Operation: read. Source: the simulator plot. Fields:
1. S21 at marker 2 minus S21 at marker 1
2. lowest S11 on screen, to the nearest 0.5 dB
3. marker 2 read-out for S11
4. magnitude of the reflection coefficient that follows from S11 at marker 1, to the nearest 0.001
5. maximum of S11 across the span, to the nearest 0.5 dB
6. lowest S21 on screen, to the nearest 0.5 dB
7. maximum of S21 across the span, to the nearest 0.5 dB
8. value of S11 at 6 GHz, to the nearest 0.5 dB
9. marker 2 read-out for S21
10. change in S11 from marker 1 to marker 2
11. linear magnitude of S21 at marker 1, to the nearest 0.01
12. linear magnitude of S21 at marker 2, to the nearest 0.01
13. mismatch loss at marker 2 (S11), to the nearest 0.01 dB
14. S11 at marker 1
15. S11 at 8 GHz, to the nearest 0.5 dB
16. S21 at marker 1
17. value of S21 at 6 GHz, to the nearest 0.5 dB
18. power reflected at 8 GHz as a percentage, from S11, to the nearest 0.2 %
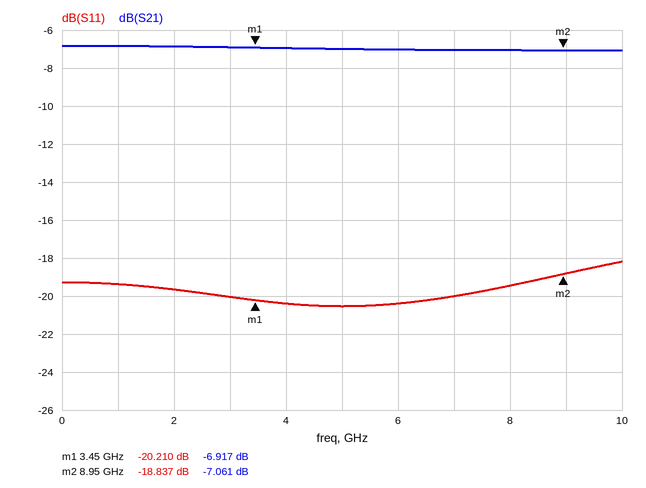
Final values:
-0.144 dB
-20.5 dB
-18.837 dB
0.098
-18.0 dB
-7.0 dB
-7.0 dB
-20.5 dB
-7.061 dB
1.373 dB
0.45
0.44
0.06 dB
-20.210 dB
-19.5 dB
-6.917 dB
-7.0 dB
1.2 %
